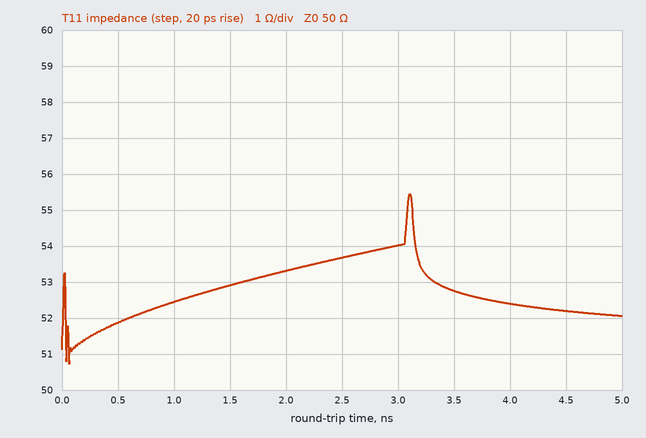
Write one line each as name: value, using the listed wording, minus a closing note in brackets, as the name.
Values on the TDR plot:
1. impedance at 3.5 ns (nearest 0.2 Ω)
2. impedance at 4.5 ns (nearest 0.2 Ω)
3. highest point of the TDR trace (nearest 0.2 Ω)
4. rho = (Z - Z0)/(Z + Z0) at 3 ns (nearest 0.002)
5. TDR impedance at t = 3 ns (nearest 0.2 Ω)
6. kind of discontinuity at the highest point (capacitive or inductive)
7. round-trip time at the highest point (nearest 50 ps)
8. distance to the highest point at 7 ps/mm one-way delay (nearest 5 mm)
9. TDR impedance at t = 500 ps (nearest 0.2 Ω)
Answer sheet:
impedance at 3.5 ns: 52.8 Ω
impedance at 4.5 ns: 52.2 Ω
highest point of the TDR trace: 55.4 Ω
rho = (Z - Z0)/(Z + Z0) at 3 ns: +0.038
TDR impedance at t = 3 ns: 54.0 Ω
kind of discontinuity at the highest point: inductive
round-trip time at the highest point: 3.10 ns
distance to the highest point at 7 ps/mm one-way delay: 220 mm
TDR impedance at t = 500 ps: 51.8 Ω
